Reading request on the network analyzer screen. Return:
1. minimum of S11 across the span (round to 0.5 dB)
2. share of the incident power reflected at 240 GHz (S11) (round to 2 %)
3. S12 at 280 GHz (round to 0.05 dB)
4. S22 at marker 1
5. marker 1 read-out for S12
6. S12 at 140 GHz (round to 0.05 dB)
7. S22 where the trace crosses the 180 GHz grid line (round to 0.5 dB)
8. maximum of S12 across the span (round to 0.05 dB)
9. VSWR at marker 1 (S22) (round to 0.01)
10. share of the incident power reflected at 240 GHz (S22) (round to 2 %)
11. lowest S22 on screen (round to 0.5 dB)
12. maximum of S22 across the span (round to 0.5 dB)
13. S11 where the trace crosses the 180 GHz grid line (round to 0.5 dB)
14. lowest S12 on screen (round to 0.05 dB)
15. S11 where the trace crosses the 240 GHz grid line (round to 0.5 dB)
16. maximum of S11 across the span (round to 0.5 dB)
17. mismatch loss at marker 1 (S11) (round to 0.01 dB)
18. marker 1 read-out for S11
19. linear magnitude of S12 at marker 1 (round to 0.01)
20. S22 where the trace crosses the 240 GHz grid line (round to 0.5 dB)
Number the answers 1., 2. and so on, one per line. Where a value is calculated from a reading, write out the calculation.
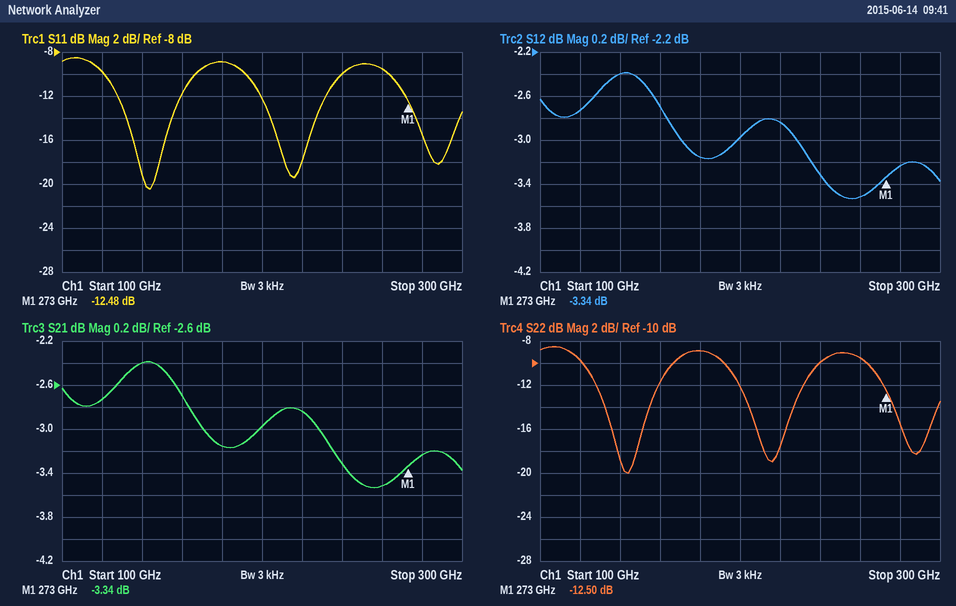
1. -20.5 dB
2. 10^(-10/10) ≈ 10 %
3. -3.25 dB
4. -12.50 dB
5. -3.34 dB
6. -2.40 dB
7. -9.0 dB
8. -2.40 dB
9. (1 + 0.2371)/(1 − 0.2371) ≈ 1.62
10. 10^(-10/10) ≈ 10 %
11. -20.0 dB
12. -8.5 dB
13. -9.0 dB
14. -3.55 dB
15. -10.0 dB
16. -8.5 dB
17. −10 log10(1 − 10^(-12.48/10)) ≈ 0.25 dB
18. -12.48 dB
19. 10^(-3.34/20) ≈ 0.68
20. -10.0 dB
